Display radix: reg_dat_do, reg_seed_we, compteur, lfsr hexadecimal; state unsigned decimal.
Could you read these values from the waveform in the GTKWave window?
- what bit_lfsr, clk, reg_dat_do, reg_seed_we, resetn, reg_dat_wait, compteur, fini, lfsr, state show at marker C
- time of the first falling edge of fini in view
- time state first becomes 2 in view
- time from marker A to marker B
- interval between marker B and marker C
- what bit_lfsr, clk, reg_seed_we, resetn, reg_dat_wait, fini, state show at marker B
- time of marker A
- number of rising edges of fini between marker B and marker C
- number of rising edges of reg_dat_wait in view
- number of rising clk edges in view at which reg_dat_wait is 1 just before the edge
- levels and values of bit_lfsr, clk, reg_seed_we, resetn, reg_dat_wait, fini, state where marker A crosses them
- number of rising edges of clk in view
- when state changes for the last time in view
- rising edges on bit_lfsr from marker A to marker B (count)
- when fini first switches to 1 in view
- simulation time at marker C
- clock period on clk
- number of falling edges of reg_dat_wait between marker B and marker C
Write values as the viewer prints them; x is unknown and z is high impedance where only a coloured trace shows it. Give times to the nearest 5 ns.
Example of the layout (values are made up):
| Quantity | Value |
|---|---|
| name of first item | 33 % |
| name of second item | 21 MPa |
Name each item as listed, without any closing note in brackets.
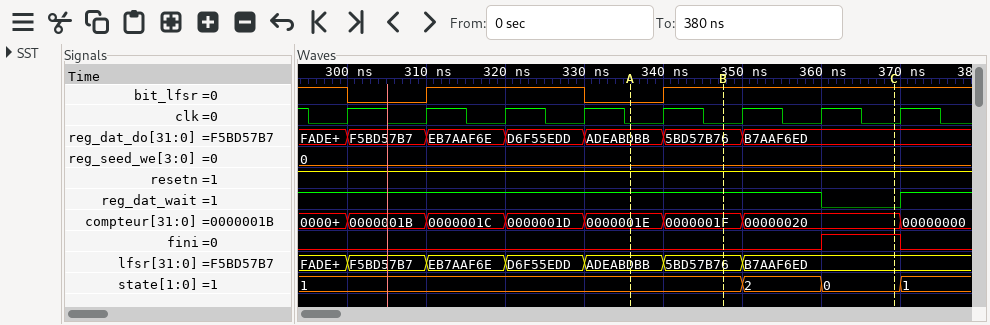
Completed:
| Quantity | Value |
|---|---|
| what bit_lfsr, clk, reg_dat_do, reg_seed_we, resetn, reg_dat_wait, compteur, fini, lfsr, state show at marker C | bit_lfsr=1, clk=0, reg_dat_do=B7AAF6ED, reg_seed_we=0, resetn=1, reg_dat_wait=0, compteur=00000020, fini=1, lfsr=B7AAF6ED, state=0 |
| time of the first falling edge of fini in view | 370 ns |
| time state first becomes 2 in view | 350 ns |
| time from marker A to marker B | 10 ns |
| interval between marker B and marker C | 20 ns |
| what bit_lfsr, clk, reg_seed_we, resetn, reg_dat_wait, fini, state show at marker B | bit_lfsr=1, clk=0, reg_seed_we=0, resetn=1, reg_dat_wait=1, fini=0, state=1 |
| time of marker A | 335 ns |
| number of rising edges of fini between marker B and marker C | 1 |
| number of rising edges of reg_dat_wait in view | 1 |
| number of rising clk edges in view at which reg_dat_wait is 1 just before the edge | 7 |
| levels and values of bit_lfsr, clk, reg_seed_we, resetn, reg_dat_wait, fini, state where marker A crosses them | bit_lfsr=0, clk=0, reg_seed_we=0, resetn=1, reg_dat_wait=1, fini=0, state=1 |
| number of rising edges of clk in view | 8 |
| when state changes for the last time in view | 370 ns |
| rising edges on bit_lfsr from marker A to marker B | 1 |
| when fini first switches to 1 in view | 360 ns |
| simulation time at marker C | 370 ns |
| clock period on clk | 10 ns |
| number of falling edges of reg_dat_wait between marker B and marker C | 1 |
